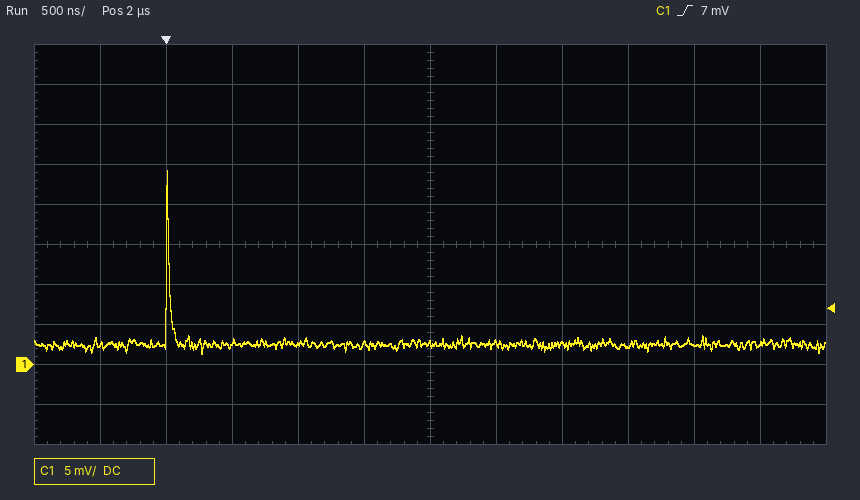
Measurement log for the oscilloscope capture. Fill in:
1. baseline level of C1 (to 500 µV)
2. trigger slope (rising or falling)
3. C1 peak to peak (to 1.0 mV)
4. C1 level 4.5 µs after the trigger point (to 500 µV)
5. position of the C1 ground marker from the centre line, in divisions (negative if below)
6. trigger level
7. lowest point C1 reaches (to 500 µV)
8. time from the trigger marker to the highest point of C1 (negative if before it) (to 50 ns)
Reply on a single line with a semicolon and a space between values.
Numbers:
2.5 mV; rising; 23.0 mV; 2.5 mV; -3.0 div; 7 mV; 1.5 mV; 0 ns
